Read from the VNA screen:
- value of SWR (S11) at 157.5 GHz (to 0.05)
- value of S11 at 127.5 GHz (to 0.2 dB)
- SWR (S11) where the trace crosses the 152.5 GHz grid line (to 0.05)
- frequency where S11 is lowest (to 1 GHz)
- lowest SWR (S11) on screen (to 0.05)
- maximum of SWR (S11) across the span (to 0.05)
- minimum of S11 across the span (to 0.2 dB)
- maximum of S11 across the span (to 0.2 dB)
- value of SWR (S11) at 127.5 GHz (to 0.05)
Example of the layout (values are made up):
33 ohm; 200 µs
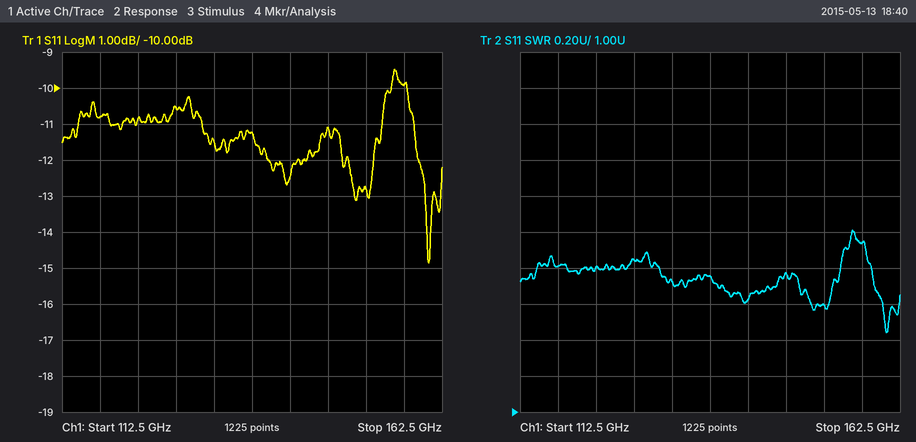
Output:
1.95; -10.6 dB; 1.60; 161 GHz; 1.45; 2.00; -14.8 dB; -9.4 dB; 1.85
